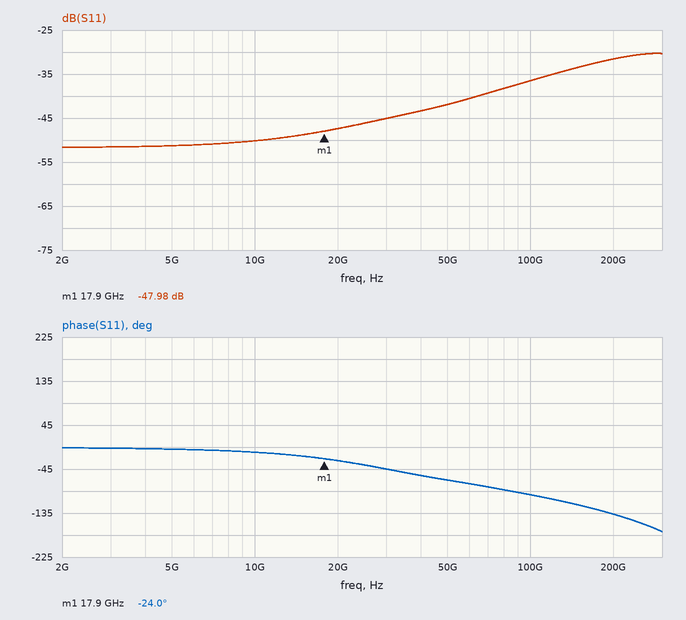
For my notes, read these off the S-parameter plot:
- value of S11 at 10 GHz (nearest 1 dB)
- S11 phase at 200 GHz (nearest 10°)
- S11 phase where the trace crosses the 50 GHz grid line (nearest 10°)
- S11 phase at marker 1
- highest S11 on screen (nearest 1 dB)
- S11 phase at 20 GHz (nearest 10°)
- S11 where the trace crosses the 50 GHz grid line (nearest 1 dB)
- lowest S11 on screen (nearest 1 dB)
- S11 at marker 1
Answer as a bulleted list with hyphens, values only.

- -50 dB
- -140°
- -70°
- -24.0°
- -30 dB
- -30°
- -42 dB
- -52 dB
- -47.98 dB
